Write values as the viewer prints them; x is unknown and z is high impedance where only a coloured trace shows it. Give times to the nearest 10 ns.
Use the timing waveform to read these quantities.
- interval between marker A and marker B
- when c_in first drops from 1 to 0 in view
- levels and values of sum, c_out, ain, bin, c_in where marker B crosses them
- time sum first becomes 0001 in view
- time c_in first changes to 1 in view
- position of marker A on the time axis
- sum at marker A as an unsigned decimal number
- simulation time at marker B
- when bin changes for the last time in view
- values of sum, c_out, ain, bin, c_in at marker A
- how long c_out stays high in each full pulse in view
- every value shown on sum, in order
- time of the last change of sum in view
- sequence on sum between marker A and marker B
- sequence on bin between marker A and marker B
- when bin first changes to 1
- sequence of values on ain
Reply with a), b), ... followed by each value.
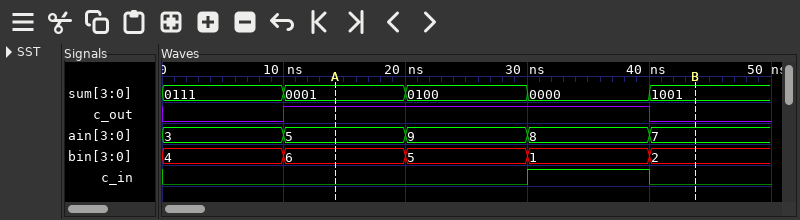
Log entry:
a) 30 ns
b) 40 ns
c) sum=1001, c_out=0, ain=7, bin=2, c_in=0
d) 10 ns
e) 30 ns
f) 10 ns
g) 1
h) 40 ns
i) 40 ns
j) sum=0001, c_out=1, ain=5, bin=6, c_in=0
k) 30 ns
l) 0111, 0001, 0100, 0000, 1001
m) 40 ns
n) 0001, 0100, 0000, 1001
o) 6, 5, 1, 2
p) 30 ns
q) 3, 5, 9, 8, 7
